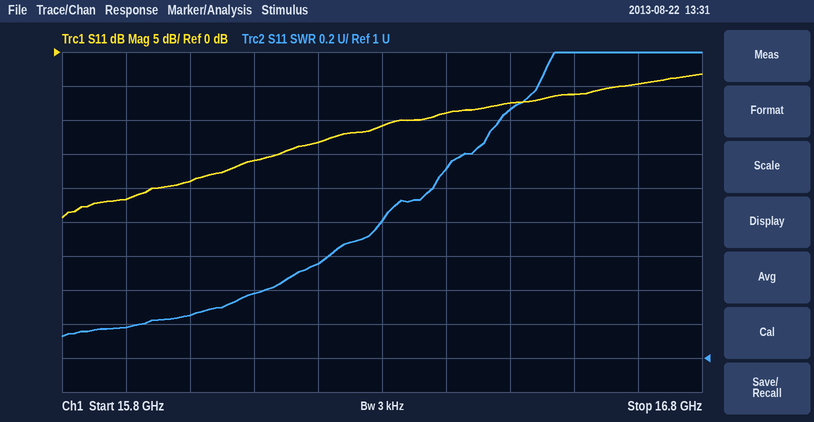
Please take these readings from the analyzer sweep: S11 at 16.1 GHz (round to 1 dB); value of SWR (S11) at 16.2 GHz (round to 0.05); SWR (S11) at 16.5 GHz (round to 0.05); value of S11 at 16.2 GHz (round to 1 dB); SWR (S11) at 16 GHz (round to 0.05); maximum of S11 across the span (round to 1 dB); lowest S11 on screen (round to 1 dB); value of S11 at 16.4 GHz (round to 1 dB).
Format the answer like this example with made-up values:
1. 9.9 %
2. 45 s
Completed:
1. -16 dB
2. 1.55
3. 2.45
4. -13 dB
5. 1.25
6. -3 dB
7. -24 dB
8. -9 dB
